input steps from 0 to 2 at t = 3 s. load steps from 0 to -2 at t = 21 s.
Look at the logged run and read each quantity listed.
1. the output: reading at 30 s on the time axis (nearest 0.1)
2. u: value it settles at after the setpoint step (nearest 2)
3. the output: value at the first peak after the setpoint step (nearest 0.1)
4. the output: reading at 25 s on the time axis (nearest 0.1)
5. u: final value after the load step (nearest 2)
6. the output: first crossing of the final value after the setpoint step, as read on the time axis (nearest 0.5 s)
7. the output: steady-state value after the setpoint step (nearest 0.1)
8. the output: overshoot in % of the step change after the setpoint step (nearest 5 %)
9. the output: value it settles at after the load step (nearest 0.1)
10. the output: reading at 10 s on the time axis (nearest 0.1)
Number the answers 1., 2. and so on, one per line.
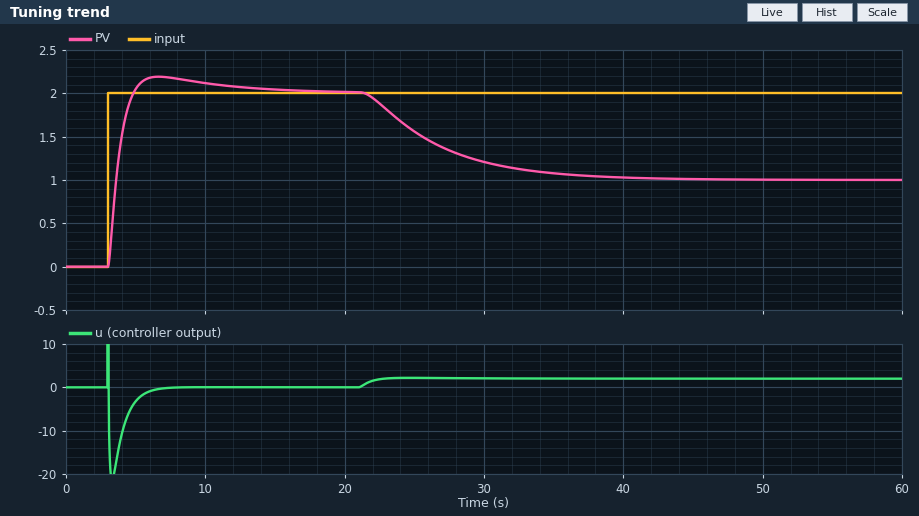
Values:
1. 1.2
2. 0
3. 2.2
4. 1.6
5. 2
6. 5.0 s
7. 2.0
8. 10 %
9. 1.0
10. 2.1
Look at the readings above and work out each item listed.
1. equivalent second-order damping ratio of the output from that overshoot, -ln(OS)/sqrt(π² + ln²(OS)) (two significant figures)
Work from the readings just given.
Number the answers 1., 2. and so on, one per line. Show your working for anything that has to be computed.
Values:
1. ln(0.1) = -2.303; 2.303 / sqrt(9.870 + 5.302) = 0.59
